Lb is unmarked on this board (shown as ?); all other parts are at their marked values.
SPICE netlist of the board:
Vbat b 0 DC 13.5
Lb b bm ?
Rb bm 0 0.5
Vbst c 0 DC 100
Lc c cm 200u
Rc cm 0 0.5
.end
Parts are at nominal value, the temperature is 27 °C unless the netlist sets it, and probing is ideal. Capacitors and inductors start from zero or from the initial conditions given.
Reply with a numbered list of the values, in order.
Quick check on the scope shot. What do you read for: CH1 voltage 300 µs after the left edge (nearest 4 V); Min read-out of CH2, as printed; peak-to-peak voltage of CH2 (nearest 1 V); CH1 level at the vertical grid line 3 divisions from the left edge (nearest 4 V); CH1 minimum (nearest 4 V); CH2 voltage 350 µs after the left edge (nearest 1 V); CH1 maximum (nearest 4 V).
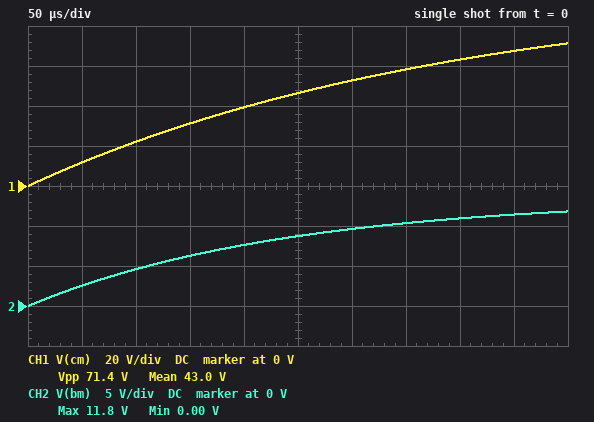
1. 52 V
2. 0.00 V
3. 12 V
4. 32 V
5. 0 V
6. 10 V
7. 72 V
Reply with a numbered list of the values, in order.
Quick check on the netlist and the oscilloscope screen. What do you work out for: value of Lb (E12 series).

1. 120 µH
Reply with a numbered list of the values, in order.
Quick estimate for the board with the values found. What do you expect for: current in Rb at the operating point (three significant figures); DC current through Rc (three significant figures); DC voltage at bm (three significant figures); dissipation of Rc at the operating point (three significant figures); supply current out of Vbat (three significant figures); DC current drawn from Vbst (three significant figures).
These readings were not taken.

1. 27.0 A
2. 200 A
3. 13.5 V
4. 20.0 kW
5. 27.0 A
6. 200 A
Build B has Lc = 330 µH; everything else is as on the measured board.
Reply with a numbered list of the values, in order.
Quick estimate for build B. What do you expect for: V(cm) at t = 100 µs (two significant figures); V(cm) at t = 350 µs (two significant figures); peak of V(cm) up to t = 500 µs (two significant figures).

1. 14 V
2. 41 V
3. 53 V
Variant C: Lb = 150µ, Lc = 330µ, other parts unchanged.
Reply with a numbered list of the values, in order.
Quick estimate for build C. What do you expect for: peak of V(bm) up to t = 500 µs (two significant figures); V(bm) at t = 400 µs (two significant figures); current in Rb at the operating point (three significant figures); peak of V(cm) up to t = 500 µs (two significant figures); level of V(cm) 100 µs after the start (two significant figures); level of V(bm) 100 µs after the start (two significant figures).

1. 11 V
2. 9.9 V
3. 27.0 A
4. 53 V
5. 14 V
6. 3.8 V
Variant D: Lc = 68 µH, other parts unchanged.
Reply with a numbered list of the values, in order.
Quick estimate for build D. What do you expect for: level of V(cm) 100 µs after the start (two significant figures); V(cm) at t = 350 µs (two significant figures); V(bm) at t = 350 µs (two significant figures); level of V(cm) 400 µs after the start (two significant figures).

1. 52 V
2. 92 V
3. 10 V
4. 95 V
